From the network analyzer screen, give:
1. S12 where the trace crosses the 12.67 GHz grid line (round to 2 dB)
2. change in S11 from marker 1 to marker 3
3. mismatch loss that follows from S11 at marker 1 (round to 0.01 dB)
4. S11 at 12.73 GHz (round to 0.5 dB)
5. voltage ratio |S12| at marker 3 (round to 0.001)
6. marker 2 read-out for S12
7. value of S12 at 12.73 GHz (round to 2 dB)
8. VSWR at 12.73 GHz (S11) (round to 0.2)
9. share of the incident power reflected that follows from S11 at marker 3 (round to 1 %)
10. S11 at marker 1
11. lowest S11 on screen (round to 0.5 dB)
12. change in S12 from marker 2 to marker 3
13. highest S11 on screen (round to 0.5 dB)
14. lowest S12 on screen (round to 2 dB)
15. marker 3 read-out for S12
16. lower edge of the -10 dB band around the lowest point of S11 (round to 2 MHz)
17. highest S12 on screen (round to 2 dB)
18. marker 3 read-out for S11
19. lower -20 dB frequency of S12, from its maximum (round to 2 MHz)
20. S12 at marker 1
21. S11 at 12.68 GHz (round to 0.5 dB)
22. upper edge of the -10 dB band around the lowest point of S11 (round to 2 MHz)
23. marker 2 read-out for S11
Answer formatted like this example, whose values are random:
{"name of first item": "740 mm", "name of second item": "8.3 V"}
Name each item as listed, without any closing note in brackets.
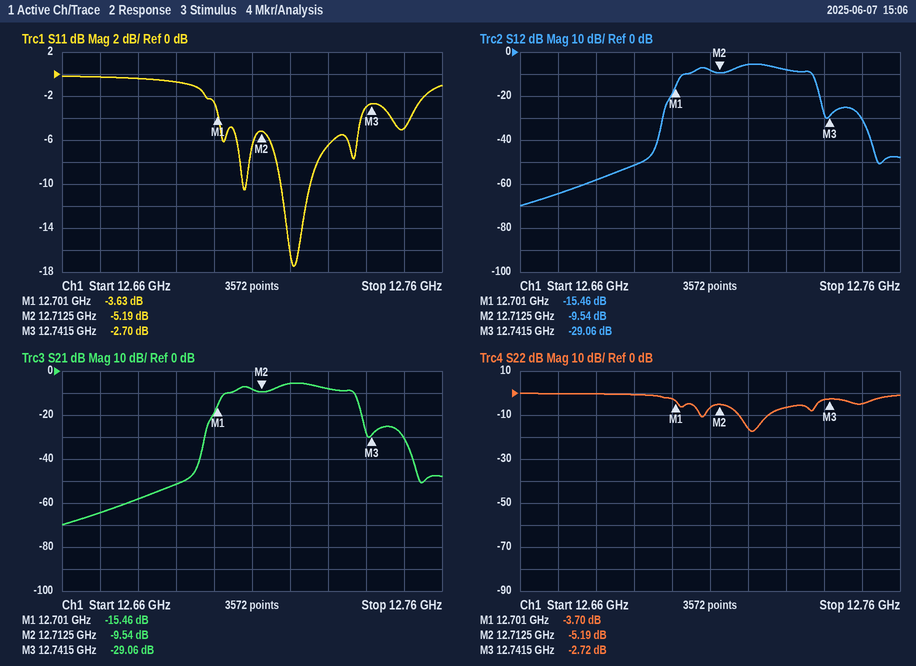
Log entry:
{"S12 where the trace crosses the 12.67 GHz grid line": "-64 dB", "change in S11 from marker 1 to marker 3": "0.93 dB", "mismatch loss that follows from S11 at marker 1": "2.47 dB", "S11 at 12.73 GHz": "-6.5 dB", "voltage ratio |S12| at marker 3": "0.035", "marker 2 read-out for S12": "-9.54 dB", "value of S12 at 12.73 GHz": "-8 dB", "VSWR at 12.73 GHz (S11)": "2.8", "share of the incident power reflected that follows from S11 at marker 3": "54 %", "S11 at marker 1": "-3.63 dB", "lowest S11 on screen": "-17.5 dB", "change in S12 from marker 2 to marker 3": "-19.52 dB", "highest S11 on screen": "0.0 dB", "lowest S12 on screen": "-70 dB", "marker 3 read-out for S12": "-29.06 dB", "lower edge of the -10 dB band around the lowest point of S11": "12.718 GHz", "highest S12 on screen": "-6 dB", "marker 3 read-out for S11": "-2.70 dB", "lower -20 dB frequency of S12, from its maximum": "12.698 GHz", "S12 at marker 1": "-15.46 dB", "S11 at 12.68 GHz": "-0.5 dB", "upper edge of the -10 dB band around the lowest point of S11": "12.726 GHz", "marker 2 read-out for S11": "-5.19 dB"}
